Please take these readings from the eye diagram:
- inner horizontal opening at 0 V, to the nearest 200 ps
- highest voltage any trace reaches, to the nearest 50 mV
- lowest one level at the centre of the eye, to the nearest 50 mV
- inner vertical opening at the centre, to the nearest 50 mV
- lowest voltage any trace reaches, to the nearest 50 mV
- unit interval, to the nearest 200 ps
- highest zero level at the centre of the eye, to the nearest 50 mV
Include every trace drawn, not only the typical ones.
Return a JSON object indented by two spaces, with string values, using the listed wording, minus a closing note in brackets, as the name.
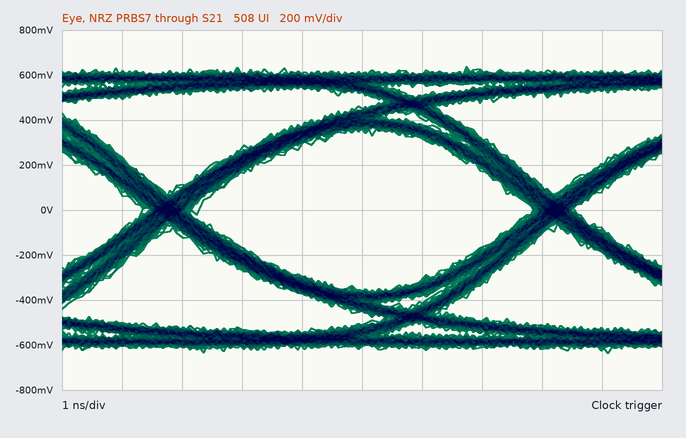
{
  "inner horizontal opening at 0 V, to the nearest 200 ps": "5.6 ns",
  "highest voltage any trace reaches, to the nearest 50 mV": "650 mV",
  "lowest one level at the centre of the eye, to the nearest 50 mV": "350 mV",
  "inner vertical opening at the centre, to the nearest 50 mV": "700 mV",
  "lowest voltage any trace reaches, to the nearest 50 mV": "-650 mV",
  "unit interval, to the nearest 200 ps": "6.4 ns",
  "highest zero level at the centre of the eye, to the nearest 50 mV": "-350 mV"
}
